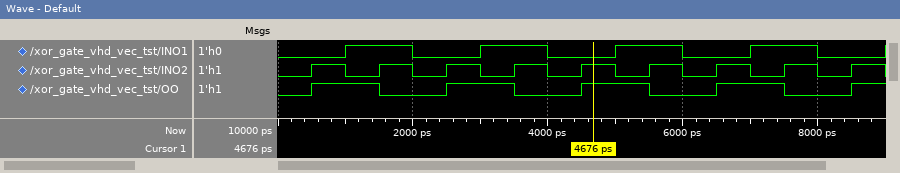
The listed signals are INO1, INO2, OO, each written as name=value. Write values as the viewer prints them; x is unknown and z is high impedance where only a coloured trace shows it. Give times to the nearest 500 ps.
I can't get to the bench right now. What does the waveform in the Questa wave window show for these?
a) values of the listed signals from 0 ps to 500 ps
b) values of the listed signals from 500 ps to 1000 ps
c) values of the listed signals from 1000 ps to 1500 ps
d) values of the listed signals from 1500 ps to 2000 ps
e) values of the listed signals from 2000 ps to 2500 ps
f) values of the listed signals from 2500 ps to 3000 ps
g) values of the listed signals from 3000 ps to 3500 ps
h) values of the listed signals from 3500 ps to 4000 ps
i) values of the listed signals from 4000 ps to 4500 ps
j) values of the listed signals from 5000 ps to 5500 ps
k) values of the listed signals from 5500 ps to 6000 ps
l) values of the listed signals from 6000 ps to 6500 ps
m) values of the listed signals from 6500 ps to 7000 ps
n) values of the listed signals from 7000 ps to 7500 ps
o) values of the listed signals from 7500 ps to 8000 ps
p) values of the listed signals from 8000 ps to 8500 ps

INO1=0, INO2=0, OO=0
INO1=0, INO2=1, OO=1
INO1=1, INO2=0, OO=1
INO1=1, INO2=1, OO=0
INO1=0, INO2=0, OO=0
INO1=0, INO2=1, OO=1
INO1=1, INO2=0, OO=1
INO1=1, INO2=1, OO=0
INO1=0, INO2=0, OO=0
INO1=1, INO2=0, OO=1
INO1=1, INO2=1, OO=0
INO1=0, INO2=0, OO=0
INO1=0, INO2=1, OO=1
INO1=1, INO2=0, OO=1
INO1=1, INO2=1, OO=0
INO1=0, INO2=0, OO=0
